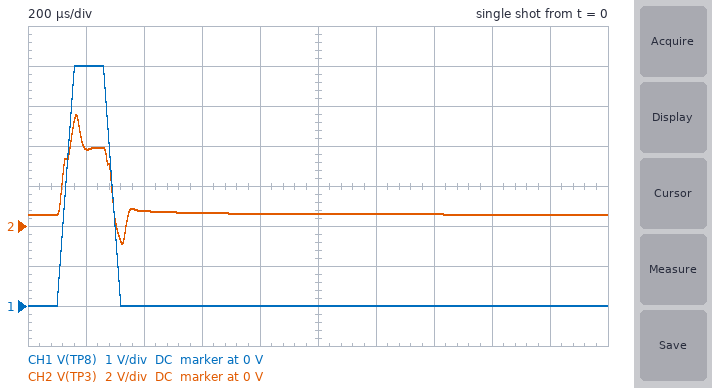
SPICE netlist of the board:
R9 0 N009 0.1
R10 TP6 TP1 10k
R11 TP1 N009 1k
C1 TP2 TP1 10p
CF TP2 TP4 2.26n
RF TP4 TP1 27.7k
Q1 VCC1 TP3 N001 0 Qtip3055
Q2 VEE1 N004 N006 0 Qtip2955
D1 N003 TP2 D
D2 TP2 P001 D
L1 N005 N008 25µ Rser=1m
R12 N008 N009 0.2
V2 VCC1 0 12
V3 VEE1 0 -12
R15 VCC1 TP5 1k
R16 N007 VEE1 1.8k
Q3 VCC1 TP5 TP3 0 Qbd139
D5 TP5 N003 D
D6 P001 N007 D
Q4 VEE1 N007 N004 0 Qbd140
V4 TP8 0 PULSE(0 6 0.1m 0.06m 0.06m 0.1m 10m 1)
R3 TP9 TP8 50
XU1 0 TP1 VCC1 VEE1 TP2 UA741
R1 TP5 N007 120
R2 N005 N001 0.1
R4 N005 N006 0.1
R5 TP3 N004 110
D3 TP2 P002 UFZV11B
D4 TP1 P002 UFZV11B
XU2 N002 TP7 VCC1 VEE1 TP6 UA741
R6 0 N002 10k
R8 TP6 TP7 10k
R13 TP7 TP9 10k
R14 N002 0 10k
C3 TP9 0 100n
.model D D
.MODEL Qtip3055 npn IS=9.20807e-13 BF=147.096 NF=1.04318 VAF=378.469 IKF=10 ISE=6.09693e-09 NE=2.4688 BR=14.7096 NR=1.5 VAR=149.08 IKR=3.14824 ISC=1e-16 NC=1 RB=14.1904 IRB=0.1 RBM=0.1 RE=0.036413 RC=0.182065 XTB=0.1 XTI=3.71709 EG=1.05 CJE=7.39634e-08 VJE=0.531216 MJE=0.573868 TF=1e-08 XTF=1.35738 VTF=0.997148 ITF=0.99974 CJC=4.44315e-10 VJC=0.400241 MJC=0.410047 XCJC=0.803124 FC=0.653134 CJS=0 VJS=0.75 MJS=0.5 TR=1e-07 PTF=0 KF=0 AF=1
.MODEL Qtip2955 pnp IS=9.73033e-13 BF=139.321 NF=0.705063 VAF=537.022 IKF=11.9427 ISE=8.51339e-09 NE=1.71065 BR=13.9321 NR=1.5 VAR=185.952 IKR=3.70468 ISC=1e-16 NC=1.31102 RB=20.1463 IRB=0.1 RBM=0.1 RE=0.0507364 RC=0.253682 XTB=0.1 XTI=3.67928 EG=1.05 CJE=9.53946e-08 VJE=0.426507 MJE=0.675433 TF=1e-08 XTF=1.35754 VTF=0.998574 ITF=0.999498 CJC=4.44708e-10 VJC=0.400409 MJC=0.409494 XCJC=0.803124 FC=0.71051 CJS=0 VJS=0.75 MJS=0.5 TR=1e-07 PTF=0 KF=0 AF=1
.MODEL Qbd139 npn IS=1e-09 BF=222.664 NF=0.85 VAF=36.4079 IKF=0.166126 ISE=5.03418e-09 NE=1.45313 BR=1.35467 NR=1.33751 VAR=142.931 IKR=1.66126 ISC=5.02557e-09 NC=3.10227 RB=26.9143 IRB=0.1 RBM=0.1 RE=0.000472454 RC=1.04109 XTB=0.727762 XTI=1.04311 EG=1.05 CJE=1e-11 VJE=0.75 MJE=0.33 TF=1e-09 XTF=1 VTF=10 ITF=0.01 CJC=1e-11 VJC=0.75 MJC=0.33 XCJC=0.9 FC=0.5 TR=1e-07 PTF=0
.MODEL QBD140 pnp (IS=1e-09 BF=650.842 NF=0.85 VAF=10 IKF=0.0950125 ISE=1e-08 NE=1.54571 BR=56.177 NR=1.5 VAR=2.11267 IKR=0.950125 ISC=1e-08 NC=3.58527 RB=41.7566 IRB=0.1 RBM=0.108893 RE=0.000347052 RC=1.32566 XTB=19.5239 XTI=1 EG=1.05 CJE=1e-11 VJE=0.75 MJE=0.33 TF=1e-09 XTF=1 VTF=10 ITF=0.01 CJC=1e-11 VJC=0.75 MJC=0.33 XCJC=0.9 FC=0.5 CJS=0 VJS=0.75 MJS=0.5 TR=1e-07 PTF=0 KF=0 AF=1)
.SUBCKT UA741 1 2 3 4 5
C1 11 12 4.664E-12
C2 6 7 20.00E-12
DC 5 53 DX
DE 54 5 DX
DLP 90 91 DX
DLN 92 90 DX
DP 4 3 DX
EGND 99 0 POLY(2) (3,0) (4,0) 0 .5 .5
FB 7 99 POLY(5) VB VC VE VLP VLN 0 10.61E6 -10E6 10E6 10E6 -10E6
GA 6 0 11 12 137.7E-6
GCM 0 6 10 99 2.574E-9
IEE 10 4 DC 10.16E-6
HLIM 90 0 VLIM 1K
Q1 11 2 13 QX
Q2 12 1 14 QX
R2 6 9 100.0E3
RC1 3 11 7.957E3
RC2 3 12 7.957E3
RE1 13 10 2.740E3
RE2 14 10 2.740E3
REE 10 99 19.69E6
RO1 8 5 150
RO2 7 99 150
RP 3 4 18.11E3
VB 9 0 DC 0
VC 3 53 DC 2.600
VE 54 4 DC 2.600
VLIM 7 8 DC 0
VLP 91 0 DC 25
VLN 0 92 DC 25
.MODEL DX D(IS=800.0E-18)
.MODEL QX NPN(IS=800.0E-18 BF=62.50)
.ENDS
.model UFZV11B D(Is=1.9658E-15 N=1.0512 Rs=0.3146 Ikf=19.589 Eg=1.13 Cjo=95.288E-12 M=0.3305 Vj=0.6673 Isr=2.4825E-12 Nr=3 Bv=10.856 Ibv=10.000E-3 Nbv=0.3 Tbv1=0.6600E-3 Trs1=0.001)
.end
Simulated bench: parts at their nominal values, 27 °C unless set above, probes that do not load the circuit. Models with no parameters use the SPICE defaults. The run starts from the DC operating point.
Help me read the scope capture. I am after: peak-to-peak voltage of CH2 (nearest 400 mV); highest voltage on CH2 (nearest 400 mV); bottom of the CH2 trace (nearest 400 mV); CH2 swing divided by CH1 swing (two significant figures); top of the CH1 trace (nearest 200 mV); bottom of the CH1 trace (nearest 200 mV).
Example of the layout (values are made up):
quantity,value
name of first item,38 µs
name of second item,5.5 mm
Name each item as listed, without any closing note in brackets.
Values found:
quantity,value
peak-to-peak voltage of CH2,6.4 V
highest voltage on CH2,5.6 V
bottom of the CH2 trace,-800 mV
CH2 swing divided by CH1 swing,1.1
top of the CH1 trace,6.0 V
bottom of the CH1 trace,0 V
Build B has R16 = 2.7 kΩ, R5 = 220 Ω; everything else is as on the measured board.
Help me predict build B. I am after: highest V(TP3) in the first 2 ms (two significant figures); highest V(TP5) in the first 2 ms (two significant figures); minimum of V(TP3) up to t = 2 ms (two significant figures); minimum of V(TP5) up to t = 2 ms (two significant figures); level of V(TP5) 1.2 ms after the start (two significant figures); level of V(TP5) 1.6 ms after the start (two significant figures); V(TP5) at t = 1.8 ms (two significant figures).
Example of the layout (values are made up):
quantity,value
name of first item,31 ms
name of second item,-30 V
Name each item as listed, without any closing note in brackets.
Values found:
quantity,value
highest V(TP3) in the first 2 ms,5.1 V
highest V(TP5) in the first 2 ms,5.5 V
minimum of V(TP3) up to t = 2 ms,-920 mV
minimum of V(TP5) up to t = 2 ms,-580 mV
level of V(TP5) 1.2 ms after the start,850 mV
level of V(TP5) 1.6 ms after the start,840 mV
V(TP5) at t = 1.8 ms,830 mV
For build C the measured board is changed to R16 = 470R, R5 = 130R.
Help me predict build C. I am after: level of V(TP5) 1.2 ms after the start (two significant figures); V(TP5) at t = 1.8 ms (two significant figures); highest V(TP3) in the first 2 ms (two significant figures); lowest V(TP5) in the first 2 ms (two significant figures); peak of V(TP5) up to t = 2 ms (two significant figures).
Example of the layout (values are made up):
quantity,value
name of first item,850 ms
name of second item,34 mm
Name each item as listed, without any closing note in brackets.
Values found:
quantity,value
level of V(TP5) 1.2 ms after the start,910 mV
V(TP5) at t = 1.8 ms,900 mV
highest V(TP3) in the first 2 ms,4.0 V
lowest V(TP5) in the first 2 ms,-510 mV
peak of V(TP5) up to t = 2 ms,4.4 V
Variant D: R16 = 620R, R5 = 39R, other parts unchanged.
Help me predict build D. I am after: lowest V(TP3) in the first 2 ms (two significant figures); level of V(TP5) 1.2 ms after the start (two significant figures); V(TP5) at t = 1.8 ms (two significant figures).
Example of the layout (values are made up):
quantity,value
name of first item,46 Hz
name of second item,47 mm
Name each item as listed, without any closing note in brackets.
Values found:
quantity,value
lowest V(TP3) in the first 2 ms,-860 mV
level of V(TP5) 1.2 ms after the start,940 mV
V(TP5) at t = 1.8 ms,930 mV
